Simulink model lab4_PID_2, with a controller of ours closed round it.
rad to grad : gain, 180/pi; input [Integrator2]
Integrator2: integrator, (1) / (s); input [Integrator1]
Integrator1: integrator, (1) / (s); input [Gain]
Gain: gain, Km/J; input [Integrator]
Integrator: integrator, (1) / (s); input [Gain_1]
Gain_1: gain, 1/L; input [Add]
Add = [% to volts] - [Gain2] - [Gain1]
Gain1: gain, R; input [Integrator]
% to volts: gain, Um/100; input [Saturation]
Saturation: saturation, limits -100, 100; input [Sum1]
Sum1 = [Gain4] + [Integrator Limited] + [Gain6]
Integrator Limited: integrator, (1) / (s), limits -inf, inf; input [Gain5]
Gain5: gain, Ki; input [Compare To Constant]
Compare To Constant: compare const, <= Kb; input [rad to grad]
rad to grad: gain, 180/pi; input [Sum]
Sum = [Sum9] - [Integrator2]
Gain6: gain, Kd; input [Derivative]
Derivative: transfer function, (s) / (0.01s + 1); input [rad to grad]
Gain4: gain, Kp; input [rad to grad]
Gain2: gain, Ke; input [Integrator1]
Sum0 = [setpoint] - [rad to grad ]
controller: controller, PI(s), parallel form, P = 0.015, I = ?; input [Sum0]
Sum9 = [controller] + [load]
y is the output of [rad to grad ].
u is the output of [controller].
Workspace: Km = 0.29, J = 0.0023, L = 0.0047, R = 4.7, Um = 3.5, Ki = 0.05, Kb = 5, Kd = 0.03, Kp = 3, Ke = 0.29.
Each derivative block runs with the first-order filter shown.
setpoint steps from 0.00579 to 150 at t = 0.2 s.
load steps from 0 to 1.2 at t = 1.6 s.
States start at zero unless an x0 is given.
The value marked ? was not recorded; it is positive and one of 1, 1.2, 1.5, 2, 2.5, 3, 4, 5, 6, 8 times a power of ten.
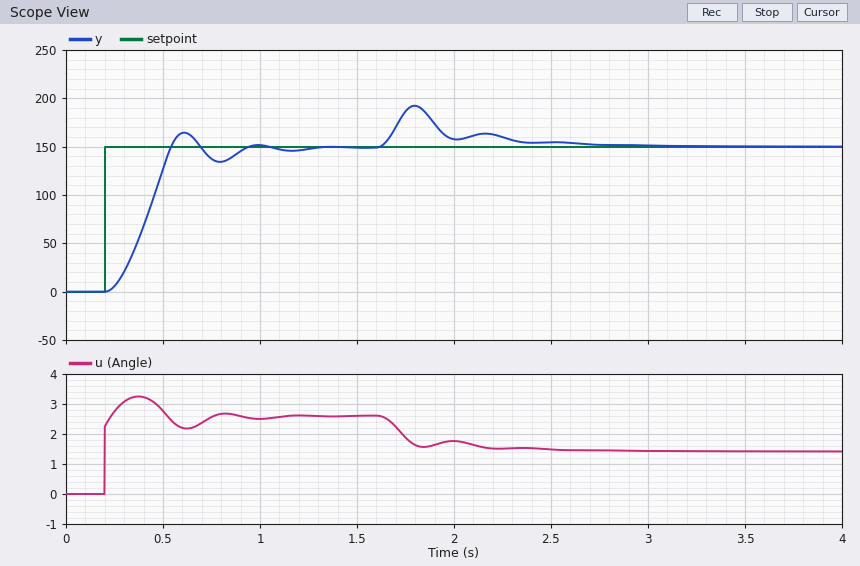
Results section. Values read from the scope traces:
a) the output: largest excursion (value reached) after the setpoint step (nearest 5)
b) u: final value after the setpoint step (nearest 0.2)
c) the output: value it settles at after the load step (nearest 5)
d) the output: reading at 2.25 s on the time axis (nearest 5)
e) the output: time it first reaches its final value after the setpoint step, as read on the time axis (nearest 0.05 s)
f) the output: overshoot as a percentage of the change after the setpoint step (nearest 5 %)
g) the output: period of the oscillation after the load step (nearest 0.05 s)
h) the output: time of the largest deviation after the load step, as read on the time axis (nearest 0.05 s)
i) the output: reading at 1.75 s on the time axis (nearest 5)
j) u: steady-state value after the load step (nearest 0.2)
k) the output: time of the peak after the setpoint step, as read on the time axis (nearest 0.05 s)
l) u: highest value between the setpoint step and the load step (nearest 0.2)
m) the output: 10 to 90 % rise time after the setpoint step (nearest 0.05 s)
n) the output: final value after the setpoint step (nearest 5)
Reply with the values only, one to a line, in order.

165
2.6
150
160
0.55 s
10 %
0.35 s
1.80 s
185
1.4
0.60 s
3.2
0.25 s
150
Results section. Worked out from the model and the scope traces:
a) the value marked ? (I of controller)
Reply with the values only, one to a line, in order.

0.08
